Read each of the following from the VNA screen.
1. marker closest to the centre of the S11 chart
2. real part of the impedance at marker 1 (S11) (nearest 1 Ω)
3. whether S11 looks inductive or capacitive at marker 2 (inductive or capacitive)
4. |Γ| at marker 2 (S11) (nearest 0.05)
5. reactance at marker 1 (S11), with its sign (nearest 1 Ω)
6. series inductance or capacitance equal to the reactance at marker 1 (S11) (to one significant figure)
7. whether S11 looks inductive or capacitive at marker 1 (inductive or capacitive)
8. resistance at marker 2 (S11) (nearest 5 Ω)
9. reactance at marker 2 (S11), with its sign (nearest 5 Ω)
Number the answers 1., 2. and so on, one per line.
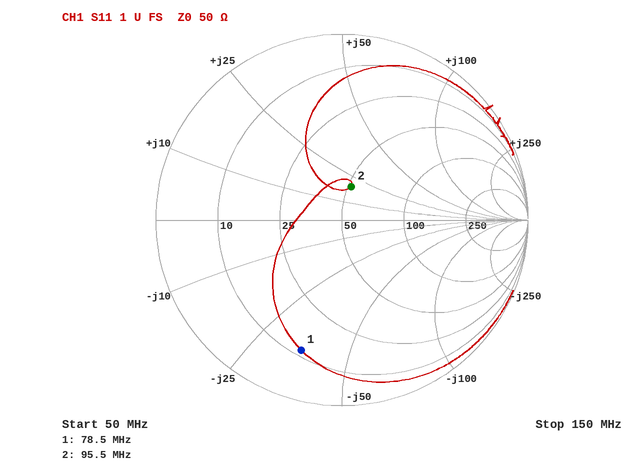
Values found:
1. marker 2
2. 12 Ω
3. inductive
4. 0.20
5. -35 Ω
6. 60 pF
7. capacitive
8. 50 Ω
9. +20 Ω
